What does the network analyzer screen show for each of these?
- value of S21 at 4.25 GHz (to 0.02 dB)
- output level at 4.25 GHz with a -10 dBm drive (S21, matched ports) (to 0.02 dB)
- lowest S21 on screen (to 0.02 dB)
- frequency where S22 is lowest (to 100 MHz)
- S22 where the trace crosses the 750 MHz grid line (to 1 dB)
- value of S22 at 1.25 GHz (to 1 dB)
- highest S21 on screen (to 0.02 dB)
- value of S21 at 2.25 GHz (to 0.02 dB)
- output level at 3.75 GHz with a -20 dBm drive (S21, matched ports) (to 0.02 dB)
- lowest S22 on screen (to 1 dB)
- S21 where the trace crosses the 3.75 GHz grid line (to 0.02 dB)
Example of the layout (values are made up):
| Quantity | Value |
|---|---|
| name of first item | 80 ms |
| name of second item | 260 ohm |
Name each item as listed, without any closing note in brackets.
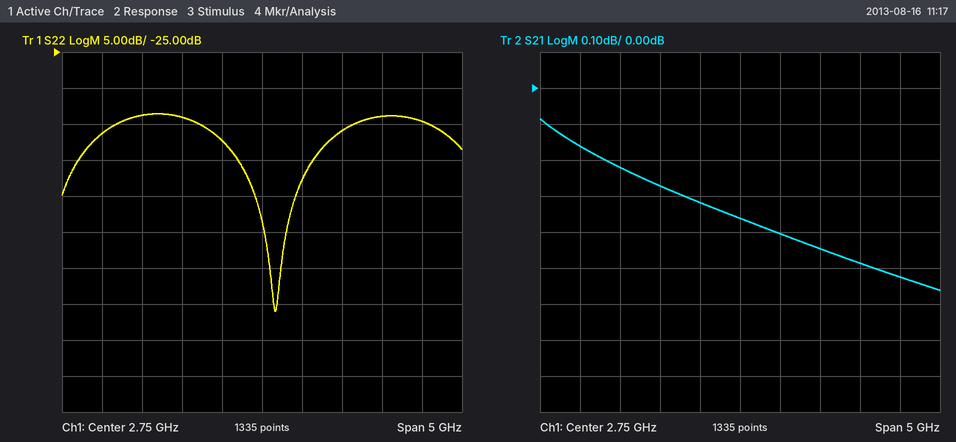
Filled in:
| Quantity | Value |
|---|---|
| value of S21 at 4.25 GHz | -0.48 dB |
| output level at 4.25 GHz with a -10 dBm drive (S21, matched ports) | -10.48 dBm |
| lowest S21 on screen | -0.56 dB |
| frequency where S22 is lowest | 2.9 GHz |
| S22 where the trace crosses the 750 MHz grid line | -36 dB |
| value of S22 at 1.25 GHz | -34 dB |
| highest S21 on screen | -0.08 dB |
| value of S21 at 2.25 GHz | -0.32 dB |
| output level at 3.75 GHz with a -20 dBm drive (S21, matched ports) | -20.44 dBm |
| lowest S22 on screen | -61 dB |
| S21 where the trace crosses the 3.75 GHz grid line | -0.44 dB |
